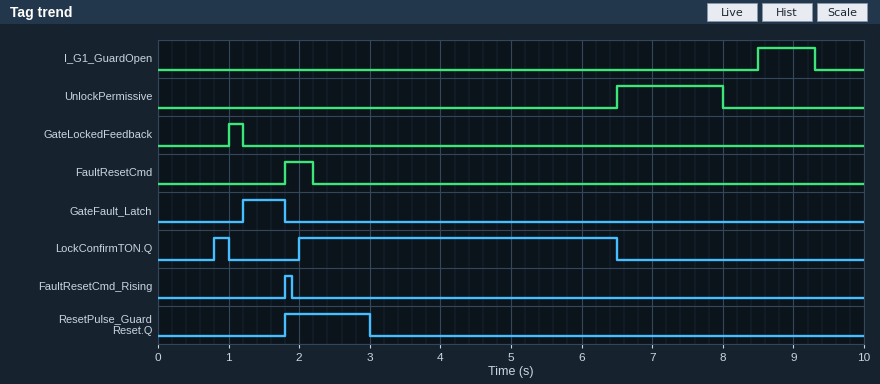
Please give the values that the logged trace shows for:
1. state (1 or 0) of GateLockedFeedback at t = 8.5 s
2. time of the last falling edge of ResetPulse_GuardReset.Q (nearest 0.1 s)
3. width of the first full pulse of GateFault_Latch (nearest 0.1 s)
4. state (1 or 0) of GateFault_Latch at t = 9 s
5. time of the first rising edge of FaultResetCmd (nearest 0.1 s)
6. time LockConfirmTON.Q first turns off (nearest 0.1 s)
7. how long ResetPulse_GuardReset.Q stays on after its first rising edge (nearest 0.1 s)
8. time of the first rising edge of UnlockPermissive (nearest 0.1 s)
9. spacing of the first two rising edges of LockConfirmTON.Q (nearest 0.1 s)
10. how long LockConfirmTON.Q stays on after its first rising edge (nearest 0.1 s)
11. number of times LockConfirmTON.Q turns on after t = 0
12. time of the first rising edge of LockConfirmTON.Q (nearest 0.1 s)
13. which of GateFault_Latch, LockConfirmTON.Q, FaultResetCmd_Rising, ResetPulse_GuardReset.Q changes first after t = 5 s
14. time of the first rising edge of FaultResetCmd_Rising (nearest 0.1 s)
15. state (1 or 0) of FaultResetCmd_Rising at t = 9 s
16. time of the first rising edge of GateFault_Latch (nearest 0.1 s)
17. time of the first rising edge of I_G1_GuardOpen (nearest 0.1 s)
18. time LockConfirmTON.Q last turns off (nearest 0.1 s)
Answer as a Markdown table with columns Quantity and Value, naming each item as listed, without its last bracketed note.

| Quantity | Value |
|---|---|
| state (1 or 0) of GateLockedFeedback at t = 8.5 s | 0 |
| time of the last falling edge of ResetPulse_GuardReset.Q | 3.0 s |
| width of the first full pulse of GateFault_Latch | 0.6 s |
| state (1 or 0) of GateFault_Latch at t = 9 s | 0 |
| time of the first rising edge of FaultResetCmd | 1.8 s |
| time LockConfirmTON.Q first turns off | 1.0 s |
| how long ResetPulse_GuardReset.Q stays on after its first rising edge | 1.2 s |
| time of the first rising edge of UnlockPermissive | 6.5 s |
| spacing of the first two rising edges of LockConfirmTON.Q | 1.2 s |
| how long LockConfirmTON.Q stays on after its first rising edge | 0.2 s |
| number of times LockConfirmTON.Q turns on after t = 0 | 2 |
| time of the first rising edge of LockConfirmTON.Q | 0.8 s |
| which of GateFault_Latch, LockConfirmTON.Q, FaultResetCmd_Rising, ResetPulse_GuardReset.Q changes first after t = 5 s | LockConfirmTON.Q |
| time of the first rising edge of FaultResetCmd_Rising | 1.8 s |
| state (1 or 0) of FaultResetCmd_Rising at t = 9 s | 0 |
| time of the first rising edge of GateFault_Latch | 1.2 s |
| time of the first rising edge of I_G1_GuardOpen | 8.5 s |
| time LockConfirmTON.Q last turns off | 6.5 s |
